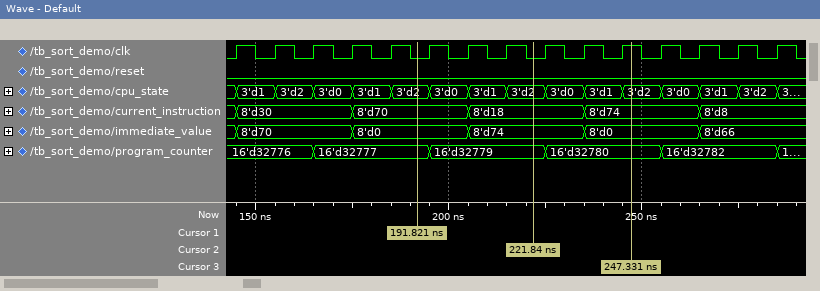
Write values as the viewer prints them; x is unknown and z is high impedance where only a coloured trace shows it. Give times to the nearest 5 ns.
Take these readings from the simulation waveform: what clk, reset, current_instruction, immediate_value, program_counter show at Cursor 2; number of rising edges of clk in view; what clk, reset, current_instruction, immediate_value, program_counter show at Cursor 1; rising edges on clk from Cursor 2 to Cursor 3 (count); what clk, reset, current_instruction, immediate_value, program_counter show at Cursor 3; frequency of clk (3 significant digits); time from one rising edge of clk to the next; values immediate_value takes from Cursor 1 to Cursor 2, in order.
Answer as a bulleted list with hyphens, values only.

- clk=0, reset=0, current_instruction=8'd18, immediate_value=8'd74, program_counter=16'd32779
- 15
- clk=0, reset=0, current_instruction=8'd70, immediate_value=8'd0, program_counter=16'd32777
- 3
- clk=1, reset=0, current_instruction=8'd74, immediate_value=8'd0, program_counter=16'd32780
- 100 MHz
- 10 ns
- 8'd0, 8'd74
